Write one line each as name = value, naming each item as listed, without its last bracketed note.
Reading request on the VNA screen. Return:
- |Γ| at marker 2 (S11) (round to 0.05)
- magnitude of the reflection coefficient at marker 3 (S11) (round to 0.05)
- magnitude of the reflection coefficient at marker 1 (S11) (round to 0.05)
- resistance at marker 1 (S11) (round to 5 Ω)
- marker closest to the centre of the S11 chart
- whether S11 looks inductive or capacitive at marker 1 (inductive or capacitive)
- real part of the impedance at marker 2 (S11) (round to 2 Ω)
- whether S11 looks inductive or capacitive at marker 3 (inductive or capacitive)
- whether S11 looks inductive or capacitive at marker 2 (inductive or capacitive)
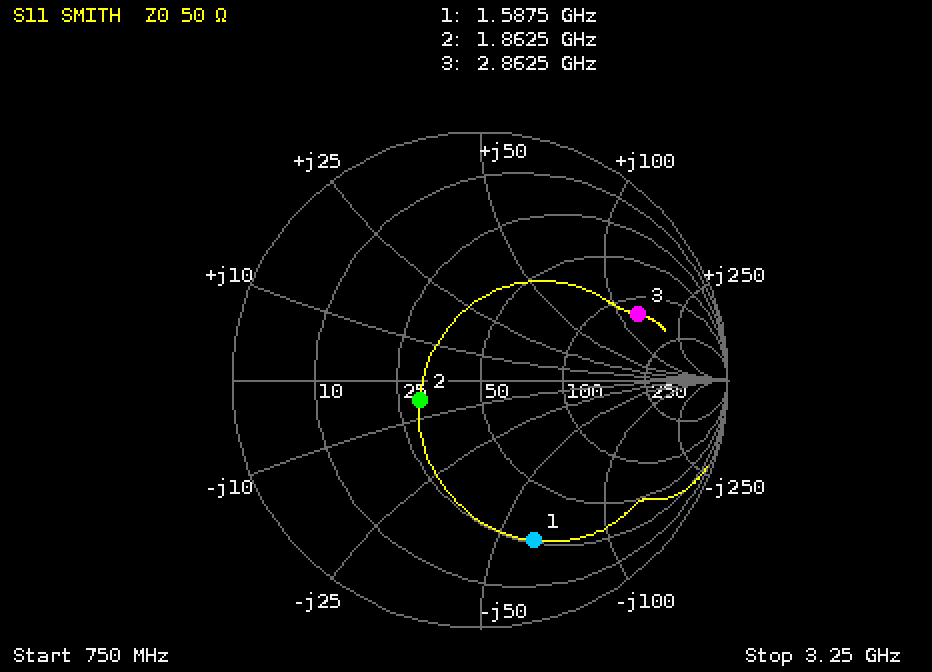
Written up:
|Γ| at marker 2 (S11) = 0.25
magnitude of the reflection coefficient at marker 3 (S11) = 0.70
magnitude of the reflection coefficient at marker 1 (S11) = 0.70
resistance at marker 1 (S11) = 25 Ω
marker closest to the centre of the S11 chart = marker 2
whether S11 looks inductive or capacitive at marker 1 = capacitive
real part of the impedance at marker 2 (S11) = 30 Ω
whether S11 looks inductive or capacitive at marker 3 = inductive
whether S11 looks inductive or capacitive at marker 2 = capacitive
